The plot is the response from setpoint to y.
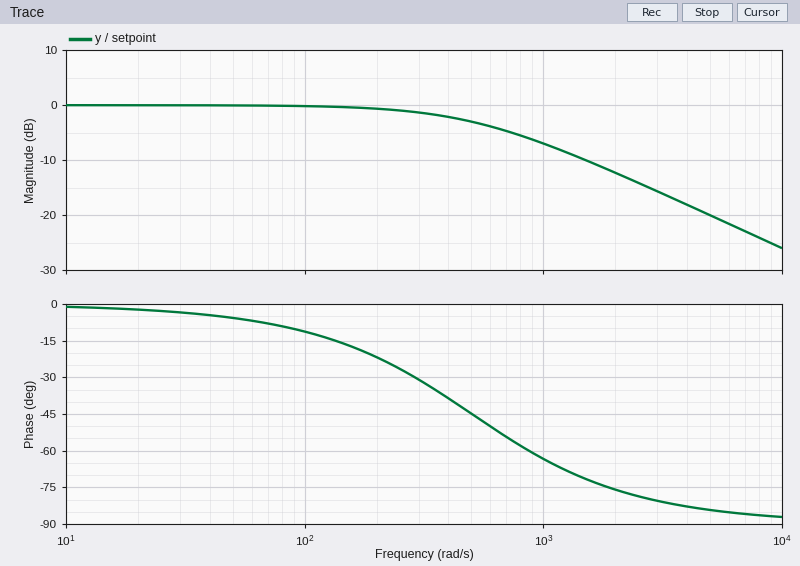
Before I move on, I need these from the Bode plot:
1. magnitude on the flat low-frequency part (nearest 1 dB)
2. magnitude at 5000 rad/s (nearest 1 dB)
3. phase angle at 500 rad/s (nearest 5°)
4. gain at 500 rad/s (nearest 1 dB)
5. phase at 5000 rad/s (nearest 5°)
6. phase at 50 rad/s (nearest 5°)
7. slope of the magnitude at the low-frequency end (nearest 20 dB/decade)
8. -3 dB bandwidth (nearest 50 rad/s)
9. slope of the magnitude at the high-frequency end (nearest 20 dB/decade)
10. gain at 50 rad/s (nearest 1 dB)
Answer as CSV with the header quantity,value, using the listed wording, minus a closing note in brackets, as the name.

quantity,value
magnitude on the flat low-frequency part,0 dB
magnitude at 5000 rad/s,-20 dB
phase angle at 500 rad/s,-45°
gain at 500 rad/s,-3 dB
phase at 5000 rad/s,-85°
phase at 50 rad/s,-5°
slope of the magnitude at the low-frequency end,0 dB/decade
-3 dB bandwidth,500 rad/s
slope of the magnitude at the high-frequency end,-20 dB/decade
gain at 50 rad/s,0 dB
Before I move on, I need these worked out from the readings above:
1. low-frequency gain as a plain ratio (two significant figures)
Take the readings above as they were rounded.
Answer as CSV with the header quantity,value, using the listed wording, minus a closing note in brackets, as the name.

quantity,value
low-frequency gain as a plain ratio,1.0
